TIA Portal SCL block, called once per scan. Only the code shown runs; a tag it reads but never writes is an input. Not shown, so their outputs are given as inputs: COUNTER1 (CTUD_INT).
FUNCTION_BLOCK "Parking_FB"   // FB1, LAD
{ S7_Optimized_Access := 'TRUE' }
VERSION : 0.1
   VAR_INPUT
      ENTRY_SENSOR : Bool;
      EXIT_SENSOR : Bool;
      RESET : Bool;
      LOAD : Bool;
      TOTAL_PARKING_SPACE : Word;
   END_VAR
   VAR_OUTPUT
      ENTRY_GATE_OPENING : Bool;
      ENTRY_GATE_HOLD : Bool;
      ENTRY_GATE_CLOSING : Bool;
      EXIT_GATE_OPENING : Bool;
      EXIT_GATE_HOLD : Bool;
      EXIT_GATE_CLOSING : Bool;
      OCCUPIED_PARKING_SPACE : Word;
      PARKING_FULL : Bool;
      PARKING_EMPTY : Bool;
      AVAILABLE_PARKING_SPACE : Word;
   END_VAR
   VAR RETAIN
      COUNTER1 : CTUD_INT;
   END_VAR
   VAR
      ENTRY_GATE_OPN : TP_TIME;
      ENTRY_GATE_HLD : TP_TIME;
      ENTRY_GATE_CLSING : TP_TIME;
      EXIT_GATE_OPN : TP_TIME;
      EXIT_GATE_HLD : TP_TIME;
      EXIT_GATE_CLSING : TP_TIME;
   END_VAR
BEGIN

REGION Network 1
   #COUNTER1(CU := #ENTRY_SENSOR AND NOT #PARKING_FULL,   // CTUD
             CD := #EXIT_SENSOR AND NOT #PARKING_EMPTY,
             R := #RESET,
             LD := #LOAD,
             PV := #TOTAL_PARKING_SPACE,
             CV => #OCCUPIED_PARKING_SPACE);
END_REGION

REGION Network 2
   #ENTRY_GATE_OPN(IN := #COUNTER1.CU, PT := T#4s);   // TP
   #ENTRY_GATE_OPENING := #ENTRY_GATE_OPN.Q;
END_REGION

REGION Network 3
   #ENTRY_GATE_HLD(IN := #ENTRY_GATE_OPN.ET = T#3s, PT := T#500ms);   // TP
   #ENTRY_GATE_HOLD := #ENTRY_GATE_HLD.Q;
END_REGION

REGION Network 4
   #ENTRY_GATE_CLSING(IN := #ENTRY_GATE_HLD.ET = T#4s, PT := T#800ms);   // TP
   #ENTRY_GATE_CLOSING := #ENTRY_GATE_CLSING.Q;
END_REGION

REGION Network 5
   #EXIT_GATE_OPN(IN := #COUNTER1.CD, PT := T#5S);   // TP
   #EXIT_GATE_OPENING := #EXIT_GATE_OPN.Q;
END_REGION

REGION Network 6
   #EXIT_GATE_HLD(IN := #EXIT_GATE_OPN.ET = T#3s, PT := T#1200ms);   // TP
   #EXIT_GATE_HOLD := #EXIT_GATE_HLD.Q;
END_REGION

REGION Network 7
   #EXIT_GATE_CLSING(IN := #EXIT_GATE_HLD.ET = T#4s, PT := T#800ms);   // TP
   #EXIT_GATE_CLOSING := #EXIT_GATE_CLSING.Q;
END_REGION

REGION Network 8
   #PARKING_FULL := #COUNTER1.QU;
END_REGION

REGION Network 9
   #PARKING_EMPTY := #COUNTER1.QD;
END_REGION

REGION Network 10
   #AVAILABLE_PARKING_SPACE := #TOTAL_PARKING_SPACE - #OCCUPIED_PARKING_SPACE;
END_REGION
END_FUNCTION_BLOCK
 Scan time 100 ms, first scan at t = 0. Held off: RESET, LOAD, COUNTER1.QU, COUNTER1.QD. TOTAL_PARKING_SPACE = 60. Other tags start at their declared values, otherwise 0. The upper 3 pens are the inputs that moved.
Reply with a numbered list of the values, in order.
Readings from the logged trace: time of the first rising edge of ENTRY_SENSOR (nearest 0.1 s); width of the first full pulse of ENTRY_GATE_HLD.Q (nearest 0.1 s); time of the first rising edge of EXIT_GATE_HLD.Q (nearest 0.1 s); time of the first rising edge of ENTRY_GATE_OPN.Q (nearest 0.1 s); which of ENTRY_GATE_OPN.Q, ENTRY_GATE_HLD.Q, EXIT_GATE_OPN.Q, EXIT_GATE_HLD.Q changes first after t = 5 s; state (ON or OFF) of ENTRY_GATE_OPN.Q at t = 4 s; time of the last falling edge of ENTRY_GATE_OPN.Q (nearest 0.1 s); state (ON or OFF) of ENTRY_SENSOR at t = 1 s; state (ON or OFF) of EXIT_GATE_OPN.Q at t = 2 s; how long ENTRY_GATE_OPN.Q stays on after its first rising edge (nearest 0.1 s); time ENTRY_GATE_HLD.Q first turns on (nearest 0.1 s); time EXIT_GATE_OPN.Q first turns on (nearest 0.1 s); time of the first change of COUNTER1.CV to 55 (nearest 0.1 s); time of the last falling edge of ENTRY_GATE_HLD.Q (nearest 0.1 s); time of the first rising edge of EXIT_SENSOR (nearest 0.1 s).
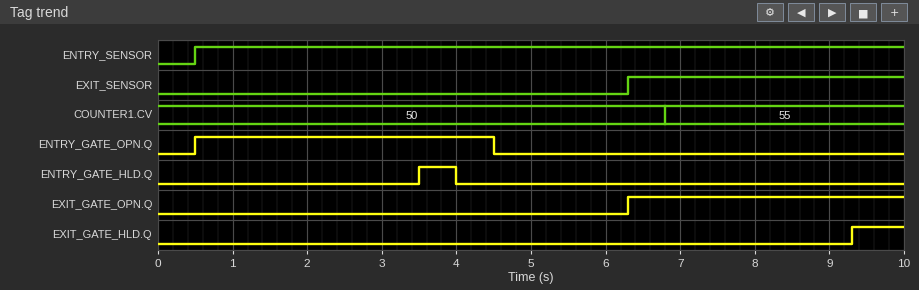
1. 0.5 s
2. 0.5 s
3. 9.3 s
4. 0.5 s
5. EXIT_GATE_OPN.Q
6. ON
7. 4.5 s
8. ON
9. OFF
10. 4.0 s
11. 3.5 s
12. 6.3 s
13. 6.8 s
14. 4.0 s
15. 6.3 s
